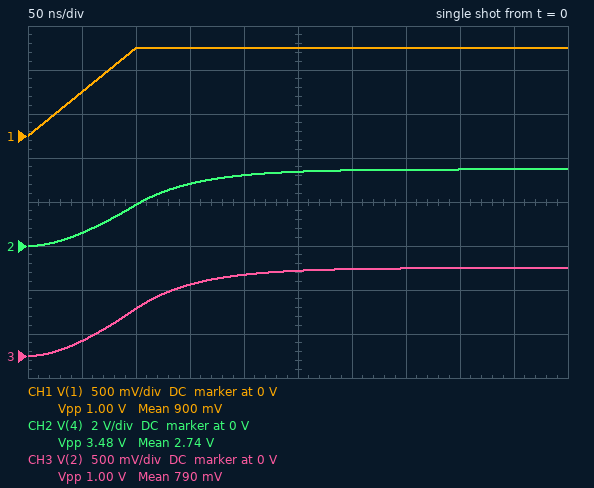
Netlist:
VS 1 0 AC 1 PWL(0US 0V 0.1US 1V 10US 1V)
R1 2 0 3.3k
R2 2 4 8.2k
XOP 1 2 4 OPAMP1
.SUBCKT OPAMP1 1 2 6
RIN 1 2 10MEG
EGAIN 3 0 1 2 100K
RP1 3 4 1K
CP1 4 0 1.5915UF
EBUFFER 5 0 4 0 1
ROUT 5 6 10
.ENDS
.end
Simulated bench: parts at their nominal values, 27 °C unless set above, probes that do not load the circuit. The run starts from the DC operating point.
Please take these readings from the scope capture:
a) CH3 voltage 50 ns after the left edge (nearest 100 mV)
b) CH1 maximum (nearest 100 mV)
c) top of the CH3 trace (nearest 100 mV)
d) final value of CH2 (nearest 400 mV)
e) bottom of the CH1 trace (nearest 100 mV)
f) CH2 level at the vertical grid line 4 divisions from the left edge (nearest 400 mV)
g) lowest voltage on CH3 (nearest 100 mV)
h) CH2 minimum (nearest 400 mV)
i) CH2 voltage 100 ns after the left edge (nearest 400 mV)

200 mV
1.0 V
1.0 V
3.6 V
0 V
3.2 V
0 V
0 V
2.0 V
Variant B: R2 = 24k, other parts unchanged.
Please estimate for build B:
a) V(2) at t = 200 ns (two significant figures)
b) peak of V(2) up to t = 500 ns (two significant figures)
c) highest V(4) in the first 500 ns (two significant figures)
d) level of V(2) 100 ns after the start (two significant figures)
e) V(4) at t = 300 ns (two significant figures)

670 mV
970 mV
8.0 V
300 mV
7.0 V
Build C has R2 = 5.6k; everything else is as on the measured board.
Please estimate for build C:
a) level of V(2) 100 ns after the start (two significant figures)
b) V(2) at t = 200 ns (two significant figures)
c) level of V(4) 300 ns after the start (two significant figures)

610 mV
960 mV
2.7 V
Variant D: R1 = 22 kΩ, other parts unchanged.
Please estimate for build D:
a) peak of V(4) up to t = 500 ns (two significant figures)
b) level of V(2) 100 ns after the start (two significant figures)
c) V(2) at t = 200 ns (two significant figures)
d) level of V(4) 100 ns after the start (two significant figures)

1.4 V
780 mV
1.0 V
1.1 V
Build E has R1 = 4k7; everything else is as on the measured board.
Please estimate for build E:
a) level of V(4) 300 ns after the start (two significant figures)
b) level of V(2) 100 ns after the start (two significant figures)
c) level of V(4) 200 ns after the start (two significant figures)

2.7 V
610 mV
2.6 V
